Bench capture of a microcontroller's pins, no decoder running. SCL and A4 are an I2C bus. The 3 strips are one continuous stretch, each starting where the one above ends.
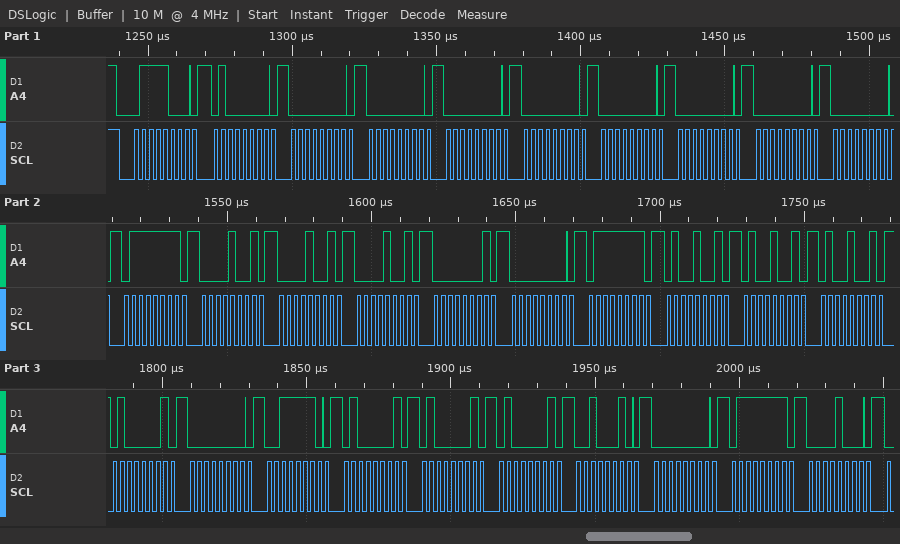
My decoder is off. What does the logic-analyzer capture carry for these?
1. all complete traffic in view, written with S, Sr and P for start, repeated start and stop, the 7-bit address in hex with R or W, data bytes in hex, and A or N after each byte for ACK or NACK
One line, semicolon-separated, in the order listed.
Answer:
S 3CW A 40 A 00 A 00 A 00 A 00 A 00 A 00 A 00 A 00 A 7F A 09 A 09 A 09 A 01 A 00 A 7F A 49 A 49 A 49 A 41 A 00 A 3E A 41 A 41 A 41 A 22 A 00 A 7F A 08 A
